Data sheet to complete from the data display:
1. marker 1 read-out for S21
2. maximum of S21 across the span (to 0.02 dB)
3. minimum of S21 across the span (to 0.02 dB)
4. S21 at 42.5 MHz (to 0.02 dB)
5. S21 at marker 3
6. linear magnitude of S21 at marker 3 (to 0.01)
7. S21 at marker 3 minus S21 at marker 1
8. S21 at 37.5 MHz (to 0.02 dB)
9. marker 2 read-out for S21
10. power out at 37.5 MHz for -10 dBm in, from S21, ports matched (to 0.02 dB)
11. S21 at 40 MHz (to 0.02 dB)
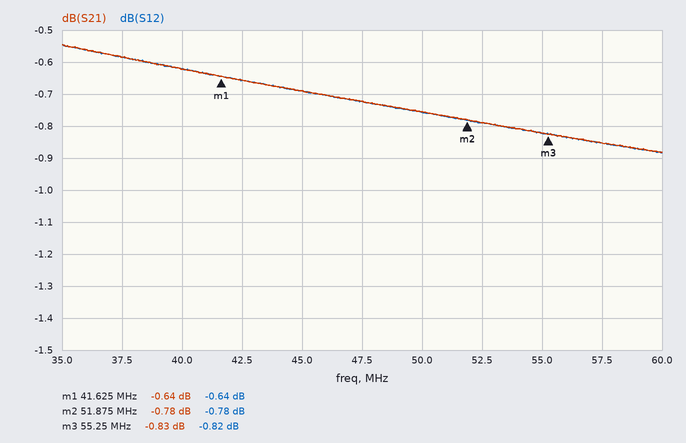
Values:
-0.64 dB
-0.54 dB
-0.88 dB
-0.66 dB
-0.83 dB
0.91
-0.19 dB
-0.58 dB
-0.78 dB
-10.58 dBm
-0.62 dB
